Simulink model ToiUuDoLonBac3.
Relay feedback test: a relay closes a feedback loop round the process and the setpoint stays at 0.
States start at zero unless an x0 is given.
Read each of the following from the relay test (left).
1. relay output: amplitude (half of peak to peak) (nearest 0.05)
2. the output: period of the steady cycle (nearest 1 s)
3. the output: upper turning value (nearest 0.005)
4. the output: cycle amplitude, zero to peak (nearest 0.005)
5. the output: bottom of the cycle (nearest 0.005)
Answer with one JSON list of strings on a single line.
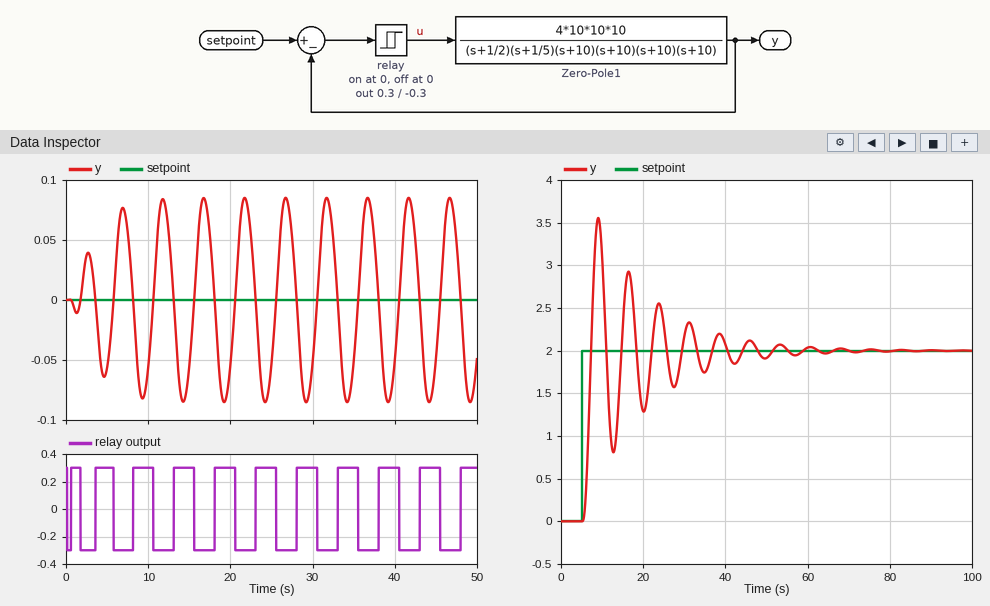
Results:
["0.30", "5 s", "0.085", "0.085", "-0.085"]
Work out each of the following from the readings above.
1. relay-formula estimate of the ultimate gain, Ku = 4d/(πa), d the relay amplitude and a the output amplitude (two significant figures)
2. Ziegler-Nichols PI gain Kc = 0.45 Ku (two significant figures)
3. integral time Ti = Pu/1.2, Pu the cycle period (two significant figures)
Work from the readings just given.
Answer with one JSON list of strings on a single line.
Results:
["4.5", "2.0", "4.2 s"]
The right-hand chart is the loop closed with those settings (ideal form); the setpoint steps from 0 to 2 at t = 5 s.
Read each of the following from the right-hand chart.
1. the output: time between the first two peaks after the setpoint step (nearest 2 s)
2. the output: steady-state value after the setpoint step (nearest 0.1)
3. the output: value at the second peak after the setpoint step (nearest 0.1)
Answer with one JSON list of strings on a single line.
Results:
["8 s", "2.0", "2.9"]
